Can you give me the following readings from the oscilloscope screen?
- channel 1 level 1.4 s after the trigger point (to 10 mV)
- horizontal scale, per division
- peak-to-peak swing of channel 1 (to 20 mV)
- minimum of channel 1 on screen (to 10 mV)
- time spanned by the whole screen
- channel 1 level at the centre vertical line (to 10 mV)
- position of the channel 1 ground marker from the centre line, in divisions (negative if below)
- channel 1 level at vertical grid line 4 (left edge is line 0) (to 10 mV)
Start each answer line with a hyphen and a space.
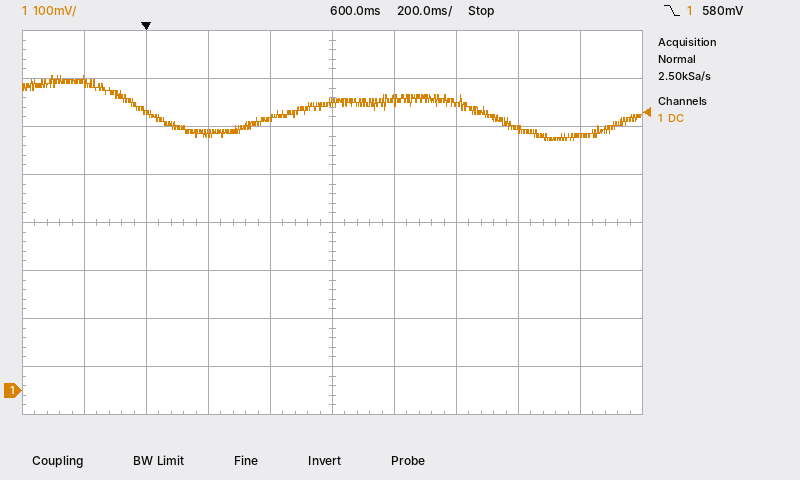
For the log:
- 530 mV
- 200 ms
- 140 mV
- 520 mV
- 2 s
- 600 mV
- -3.5 div
- 570 mV
